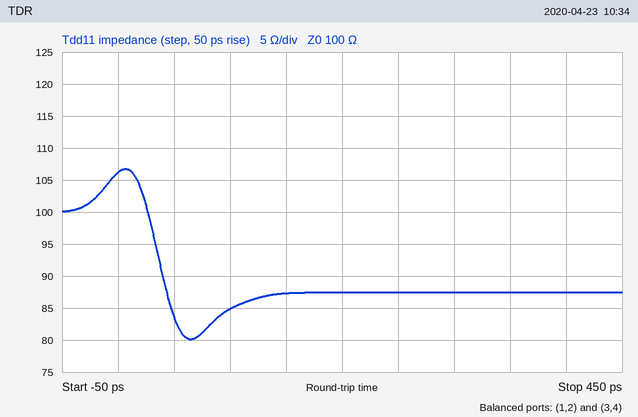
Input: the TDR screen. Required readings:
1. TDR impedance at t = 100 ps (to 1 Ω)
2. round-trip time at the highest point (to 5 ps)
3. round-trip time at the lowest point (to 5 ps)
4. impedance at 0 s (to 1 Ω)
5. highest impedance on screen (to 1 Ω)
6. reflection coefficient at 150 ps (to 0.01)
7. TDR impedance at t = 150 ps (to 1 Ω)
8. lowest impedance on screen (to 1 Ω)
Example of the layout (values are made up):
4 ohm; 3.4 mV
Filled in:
85 Ω; 5 ps; 65 ps; 106 Ω; 107 Ω; -0.07; 87 Ω; 80 Ω
